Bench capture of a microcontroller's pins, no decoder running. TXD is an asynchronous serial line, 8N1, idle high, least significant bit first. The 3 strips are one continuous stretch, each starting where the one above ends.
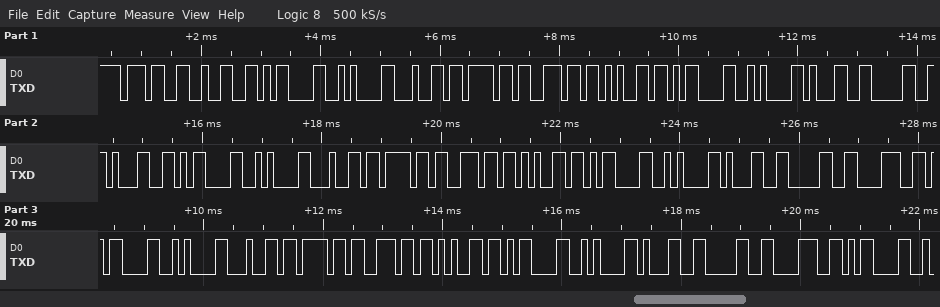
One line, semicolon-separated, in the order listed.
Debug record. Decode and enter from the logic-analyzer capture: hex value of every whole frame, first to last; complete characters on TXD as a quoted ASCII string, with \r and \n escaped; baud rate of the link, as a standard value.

0x37 0x32 0x0D 0x0A 0x64 0x6F 0x6E 0x65 0x0D 0x0A 0x31 0x30 0x31 0x0D 0x0A 0x64 0x6F 0x6E 0x65 0x0D 0x0A 0x31 0x30 0x38 0x0D 0x0A 0x64 0x6F 0x6E 0x65 0x0D 0x0A 0x31 0x30 0x38 0x0D; "72\r\ndone\r\n101\r\ndone\r\n108\r\ndone\r\n108\r"; 9600 baud
